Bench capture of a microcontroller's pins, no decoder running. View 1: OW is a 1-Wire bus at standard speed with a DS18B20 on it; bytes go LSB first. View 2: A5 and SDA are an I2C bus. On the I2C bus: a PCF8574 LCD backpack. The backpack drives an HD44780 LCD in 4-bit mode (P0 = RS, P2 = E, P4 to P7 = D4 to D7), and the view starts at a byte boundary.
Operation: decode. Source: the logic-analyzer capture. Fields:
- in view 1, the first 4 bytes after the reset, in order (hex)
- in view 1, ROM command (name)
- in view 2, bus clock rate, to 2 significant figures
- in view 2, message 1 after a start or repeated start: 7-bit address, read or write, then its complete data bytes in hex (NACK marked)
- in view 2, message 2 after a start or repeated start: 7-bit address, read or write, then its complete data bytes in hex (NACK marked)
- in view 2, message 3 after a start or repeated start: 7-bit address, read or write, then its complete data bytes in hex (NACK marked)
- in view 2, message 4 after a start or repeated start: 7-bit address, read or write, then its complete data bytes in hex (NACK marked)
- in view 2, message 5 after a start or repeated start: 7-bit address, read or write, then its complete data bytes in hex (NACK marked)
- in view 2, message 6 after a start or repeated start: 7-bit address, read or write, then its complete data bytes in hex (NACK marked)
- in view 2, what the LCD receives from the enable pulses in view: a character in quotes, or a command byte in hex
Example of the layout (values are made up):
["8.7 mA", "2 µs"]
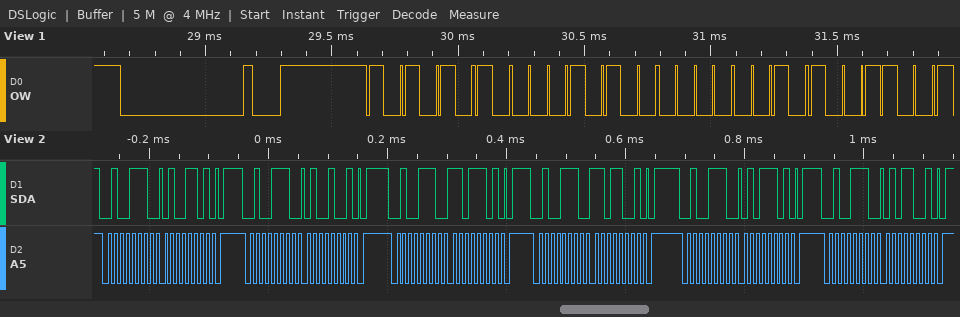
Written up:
["55 28 40 99", "Match ROM", "100 kHz", "0x27 write: 4D", "0x27 write: 49", "0x27 write: DD", "0x27 write: D9", "0x27 write: 5D", "0x27 write: 59", "'M'"]
